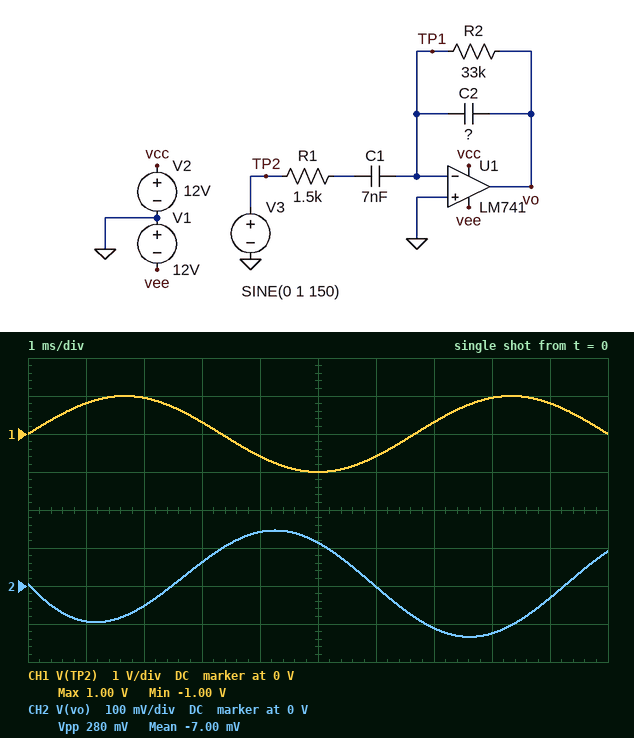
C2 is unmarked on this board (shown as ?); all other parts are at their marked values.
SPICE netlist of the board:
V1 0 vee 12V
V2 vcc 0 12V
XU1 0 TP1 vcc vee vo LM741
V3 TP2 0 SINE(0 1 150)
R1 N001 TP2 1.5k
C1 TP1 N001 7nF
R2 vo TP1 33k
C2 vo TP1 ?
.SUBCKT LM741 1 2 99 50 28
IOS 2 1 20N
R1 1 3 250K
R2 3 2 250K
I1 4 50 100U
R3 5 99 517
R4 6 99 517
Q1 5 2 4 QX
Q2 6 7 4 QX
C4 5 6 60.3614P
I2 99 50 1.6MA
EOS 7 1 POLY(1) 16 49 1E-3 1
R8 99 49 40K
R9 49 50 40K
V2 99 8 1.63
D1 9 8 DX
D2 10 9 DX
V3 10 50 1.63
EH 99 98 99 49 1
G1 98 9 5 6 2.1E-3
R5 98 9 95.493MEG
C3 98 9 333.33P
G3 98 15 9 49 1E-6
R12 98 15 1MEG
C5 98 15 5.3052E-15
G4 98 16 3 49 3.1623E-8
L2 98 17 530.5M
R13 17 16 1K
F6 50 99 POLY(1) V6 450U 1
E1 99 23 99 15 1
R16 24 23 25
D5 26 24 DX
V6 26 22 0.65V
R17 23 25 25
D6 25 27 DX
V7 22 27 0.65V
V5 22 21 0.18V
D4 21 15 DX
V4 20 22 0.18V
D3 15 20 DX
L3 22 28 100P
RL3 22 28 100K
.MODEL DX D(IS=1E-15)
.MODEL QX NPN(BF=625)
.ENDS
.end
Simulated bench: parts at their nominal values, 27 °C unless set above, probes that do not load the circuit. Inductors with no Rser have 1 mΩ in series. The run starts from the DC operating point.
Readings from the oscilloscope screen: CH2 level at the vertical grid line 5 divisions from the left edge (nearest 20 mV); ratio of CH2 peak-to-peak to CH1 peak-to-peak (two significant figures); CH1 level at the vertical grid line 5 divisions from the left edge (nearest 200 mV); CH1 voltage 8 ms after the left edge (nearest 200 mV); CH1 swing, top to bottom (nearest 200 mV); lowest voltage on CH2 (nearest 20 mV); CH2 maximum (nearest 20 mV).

120 mV
0.14
-1.0 V
1.0 V
2.0 V
-140 mV
140 mV
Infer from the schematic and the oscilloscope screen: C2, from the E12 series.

39 nF
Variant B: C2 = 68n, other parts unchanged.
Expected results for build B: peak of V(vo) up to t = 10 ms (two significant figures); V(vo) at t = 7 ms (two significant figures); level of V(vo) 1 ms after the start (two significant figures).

100 mV
-57 mV
-61 mV
